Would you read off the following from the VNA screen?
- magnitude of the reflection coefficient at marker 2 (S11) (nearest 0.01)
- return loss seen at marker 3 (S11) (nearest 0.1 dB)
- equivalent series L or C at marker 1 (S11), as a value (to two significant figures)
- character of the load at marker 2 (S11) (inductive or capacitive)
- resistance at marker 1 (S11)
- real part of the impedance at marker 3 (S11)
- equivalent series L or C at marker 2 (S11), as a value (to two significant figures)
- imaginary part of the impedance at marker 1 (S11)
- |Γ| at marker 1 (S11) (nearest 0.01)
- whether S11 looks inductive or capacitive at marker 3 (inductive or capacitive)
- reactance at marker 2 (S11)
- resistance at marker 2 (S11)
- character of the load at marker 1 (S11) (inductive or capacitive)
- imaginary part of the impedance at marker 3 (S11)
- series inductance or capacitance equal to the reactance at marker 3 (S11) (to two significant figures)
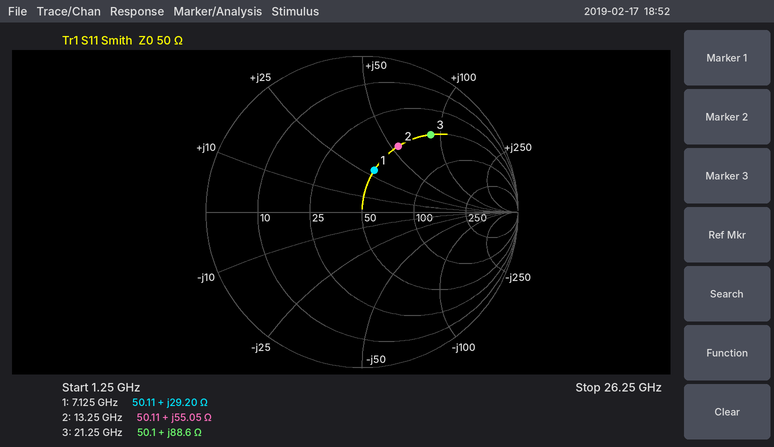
0.48
3.6 dB
650 pH
inductive
50.11 Ω
50.1 Ω
660 pH
+29.20 Ω
0.28
inductive
+55.05 Ω
50.11 Ω
inductive
+88.6 Ω
660 pH
